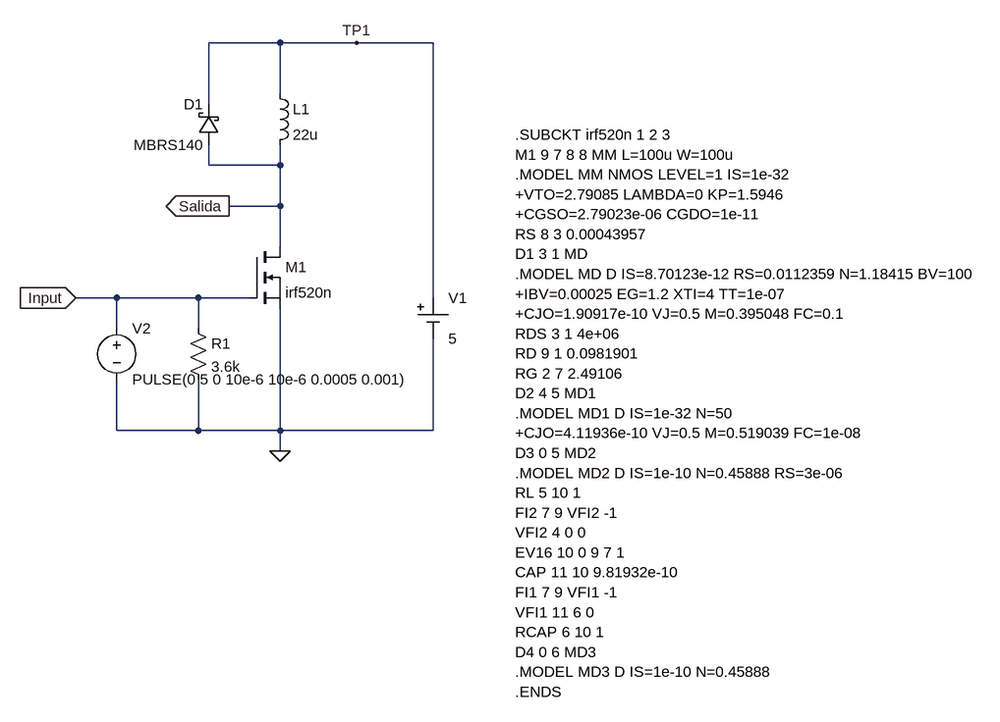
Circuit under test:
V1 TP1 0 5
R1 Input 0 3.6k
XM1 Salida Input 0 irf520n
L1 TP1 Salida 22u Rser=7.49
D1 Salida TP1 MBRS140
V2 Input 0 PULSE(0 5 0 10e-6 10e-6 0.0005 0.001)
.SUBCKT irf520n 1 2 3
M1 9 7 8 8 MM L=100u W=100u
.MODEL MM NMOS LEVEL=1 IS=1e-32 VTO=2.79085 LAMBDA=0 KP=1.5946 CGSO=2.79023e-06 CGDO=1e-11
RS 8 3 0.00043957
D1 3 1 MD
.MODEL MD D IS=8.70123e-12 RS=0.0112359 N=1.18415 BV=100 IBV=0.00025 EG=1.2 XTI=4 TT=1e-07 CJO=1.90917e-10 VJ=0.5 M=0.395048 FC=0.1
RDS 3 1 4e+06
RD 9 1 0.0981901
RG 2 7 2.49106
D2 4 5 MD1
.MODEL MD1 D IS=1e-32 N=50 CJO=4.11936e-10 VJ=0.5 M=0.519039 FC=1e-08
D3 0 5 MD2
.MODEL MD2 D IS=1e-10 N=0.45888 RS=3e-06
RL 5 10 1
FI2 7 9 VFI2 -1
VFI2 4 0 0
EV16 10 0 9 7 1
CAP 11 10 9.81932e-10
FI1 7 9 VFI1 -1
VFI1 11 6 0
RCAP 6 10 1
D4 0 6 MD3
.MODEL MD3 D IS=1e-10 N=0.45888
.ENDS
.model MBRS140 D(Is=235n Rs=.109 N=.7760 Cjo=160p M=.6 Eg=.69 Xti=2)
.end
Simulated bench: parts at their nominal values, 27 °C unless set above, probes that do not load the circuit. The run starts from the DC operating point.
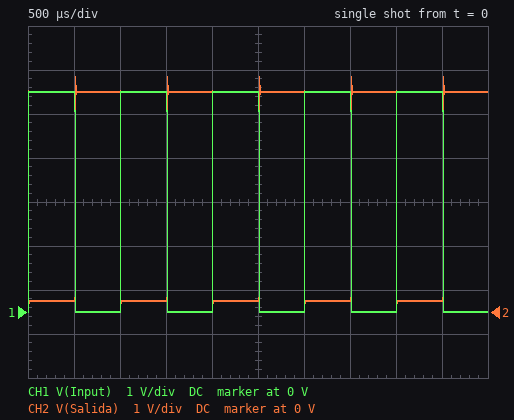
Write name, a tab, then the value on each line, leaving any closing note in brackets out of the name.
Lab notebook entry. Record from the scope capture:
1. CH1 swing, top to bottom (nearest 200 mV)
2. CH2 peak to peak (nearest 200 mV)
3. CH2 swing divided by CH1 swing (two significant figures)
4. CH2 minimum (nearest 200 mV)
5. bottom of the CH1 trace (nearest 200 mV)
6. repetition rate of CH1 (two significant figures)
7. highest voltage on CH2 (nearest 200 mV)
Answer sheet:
CH1 swing, top to bottom	5.0 V
CH2 peak to peak	5.2 V
CH2 swing divided by CH1 swing	1.0
CH2 minimum	200 mV
bottom of the CH1 trace	0 V
repetition rate of CH1	1.0 kHz
highest voltage on CH2	5.4 V
